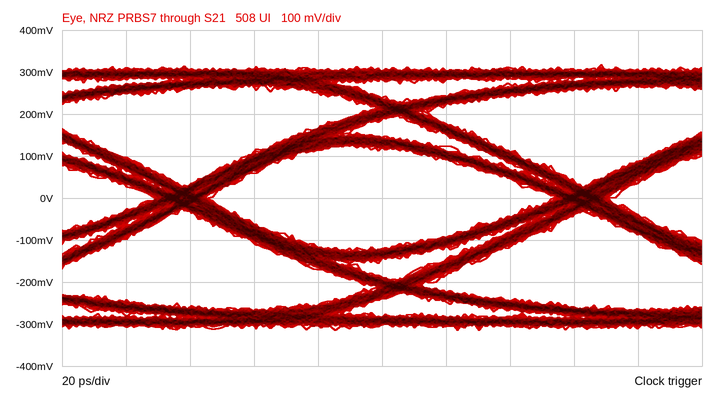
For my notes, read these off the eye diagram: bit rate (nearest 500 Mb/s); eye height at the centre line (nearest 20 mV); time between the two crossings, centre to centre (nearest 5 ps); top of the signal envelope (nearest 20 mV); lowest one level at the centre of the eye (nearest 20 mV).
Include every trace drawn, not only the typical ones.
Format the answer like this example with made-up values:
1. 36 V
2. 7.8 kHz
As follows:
1. 8.0 Gb/s
2. 240 mV
3. 125 ps
4. 320 mV
5. 120 mV
